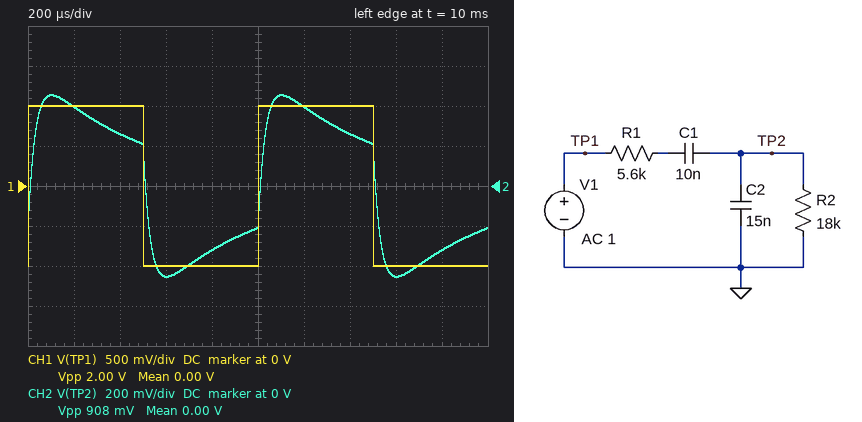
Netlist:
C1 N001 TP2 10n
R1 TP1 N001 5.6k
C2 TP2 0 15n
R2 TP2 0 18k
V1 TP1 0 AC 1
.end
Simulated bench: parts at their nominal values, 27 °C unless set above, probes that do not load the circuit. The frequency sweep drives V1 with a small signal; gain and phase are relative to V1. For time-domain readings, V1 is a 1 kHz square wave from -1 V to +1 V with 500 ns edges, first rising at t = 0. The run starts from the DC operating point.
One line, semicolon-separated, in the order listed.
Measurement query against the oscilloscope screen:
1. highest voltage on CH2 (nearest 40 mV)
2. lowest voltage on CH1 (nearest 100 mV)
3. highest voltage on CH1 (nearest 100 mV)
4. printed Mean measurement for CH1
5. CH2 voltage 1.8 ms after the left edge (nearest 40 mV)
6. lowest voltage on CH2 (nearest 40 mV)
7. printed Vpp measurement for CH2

440 mV; -1.0 V; 1.0 V; 0.00 V; -320 mV; -440 mV; 908 mV
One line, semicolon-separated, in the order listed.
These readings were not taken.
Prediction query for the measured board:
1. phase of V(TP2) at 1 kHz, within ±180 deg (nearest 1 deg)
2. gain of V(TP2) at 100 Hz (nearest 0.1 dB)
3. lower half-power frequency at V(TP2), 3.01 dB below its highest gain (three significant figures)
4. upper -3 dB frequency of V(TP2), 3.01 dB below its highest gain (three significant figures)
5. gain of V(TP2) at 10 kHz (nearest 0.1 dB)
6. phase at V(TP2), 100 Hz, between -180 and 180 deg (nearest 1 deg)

7 deg; -19.3 dB; 298 Hz; 5.62 kHz; -15.4 dB; 72 deg
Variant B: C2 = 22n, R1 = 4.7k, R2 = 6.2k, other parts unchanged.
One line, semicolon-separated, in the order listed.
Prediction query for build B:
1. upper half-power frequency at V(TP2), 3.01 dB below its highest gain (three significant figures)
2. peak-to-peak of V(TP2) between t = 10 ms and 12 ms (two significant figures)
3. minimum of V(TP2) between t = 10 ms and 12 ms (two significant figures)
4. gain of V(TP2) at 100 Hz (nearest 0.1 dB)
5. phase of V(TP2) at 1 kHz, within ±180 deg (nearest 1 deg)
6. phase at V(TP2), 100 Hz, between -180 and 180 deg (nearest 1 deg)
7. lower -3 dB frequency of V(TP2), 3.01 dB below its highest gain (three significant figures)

6.68 kHz; 750 mV; -380 mV; -28.3 dB; 26 deg; 81 deg; 591 Hz
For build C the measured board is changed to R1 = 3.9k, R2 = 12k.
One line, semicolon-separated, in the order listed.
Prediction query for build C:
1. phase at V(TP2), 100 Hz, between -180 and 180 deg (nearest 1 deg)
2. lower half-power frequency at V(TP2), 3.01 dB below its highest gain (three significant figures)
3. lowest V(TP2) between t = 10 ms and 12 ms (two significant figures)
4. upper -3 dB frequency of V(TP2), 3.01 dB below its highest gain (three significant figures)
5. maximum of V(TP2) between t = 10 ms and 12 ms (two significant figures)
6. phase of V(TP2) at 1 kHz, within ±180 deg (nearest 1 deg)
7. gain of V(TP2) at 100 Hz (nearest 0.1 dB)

78 deg; 444 Hz; -510 mV; 8.13 kHz; 510 mV; 19 deg; -22.6 dB
